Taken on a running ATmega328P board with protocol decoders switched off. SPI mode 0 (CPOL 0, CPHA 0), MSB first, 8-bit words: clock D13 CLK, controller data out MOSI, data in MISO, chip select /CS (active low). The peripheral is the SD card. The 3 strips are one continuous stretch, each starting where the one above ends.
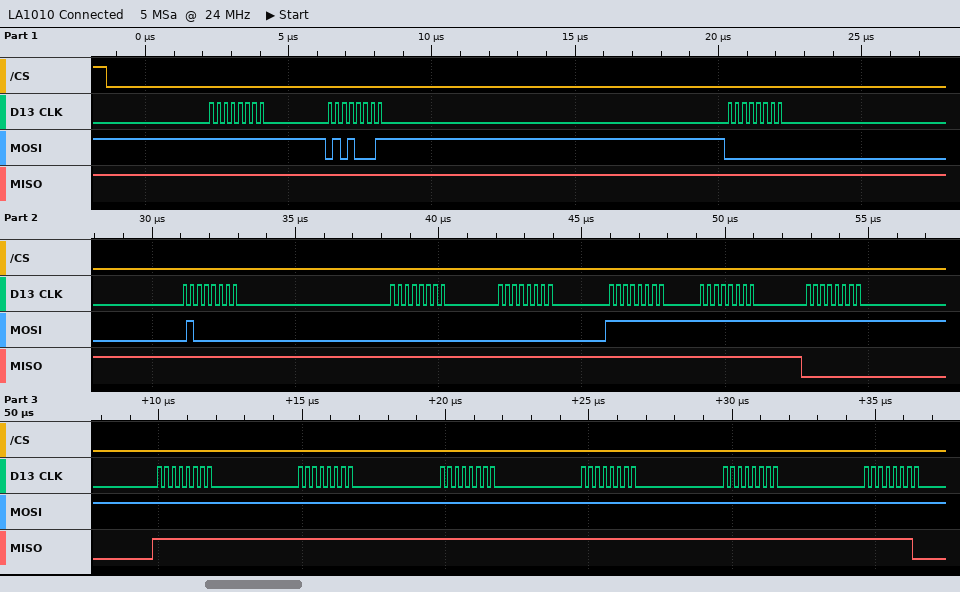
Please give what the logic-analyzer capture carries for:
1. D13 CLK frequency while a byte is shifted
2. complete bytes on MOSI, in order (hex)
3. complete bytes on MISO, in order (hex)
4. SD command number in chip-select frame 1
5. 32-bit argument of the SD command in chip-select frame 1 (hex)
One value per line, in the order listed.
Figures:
4 MHz
0xFF 0x51 0x00 0x40 0x00 0x00 0xFF 0xFF 0xFF 0xFF 0xFF 0xFF 0xFF 0xFF 0xFF
0xFF 0xFF 0xFF 0xFF 0xFF 0xFF 0xFF 0xFF 0x00 0xFF 0xFF 0xFF 0xFF 0xFF 0xFE
CMD17
0x00400000
